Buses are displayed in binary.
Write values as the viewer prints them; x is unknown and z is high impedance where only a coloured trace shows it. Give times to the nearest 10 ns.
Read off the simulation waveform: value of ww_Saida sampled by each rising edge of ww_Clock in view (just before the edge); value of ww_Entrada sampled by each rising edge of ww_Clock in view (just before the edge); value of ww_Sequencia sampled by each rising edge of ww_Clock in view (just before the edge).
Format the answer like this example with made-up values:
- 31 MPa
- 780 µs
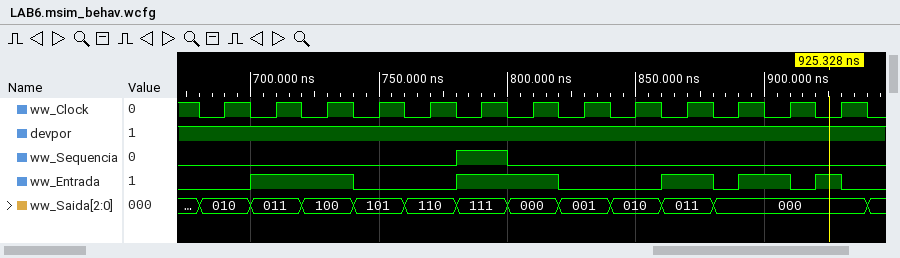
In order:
- 010, 011, 100, 101, 110, 111, 000, 001, 010, 011, 000, 000, 000
- 0 1 1 0 0 1 1 0 0 1 0 1 1
- 0 0 0 0 0 1 0 0 0 0 0 0 0
